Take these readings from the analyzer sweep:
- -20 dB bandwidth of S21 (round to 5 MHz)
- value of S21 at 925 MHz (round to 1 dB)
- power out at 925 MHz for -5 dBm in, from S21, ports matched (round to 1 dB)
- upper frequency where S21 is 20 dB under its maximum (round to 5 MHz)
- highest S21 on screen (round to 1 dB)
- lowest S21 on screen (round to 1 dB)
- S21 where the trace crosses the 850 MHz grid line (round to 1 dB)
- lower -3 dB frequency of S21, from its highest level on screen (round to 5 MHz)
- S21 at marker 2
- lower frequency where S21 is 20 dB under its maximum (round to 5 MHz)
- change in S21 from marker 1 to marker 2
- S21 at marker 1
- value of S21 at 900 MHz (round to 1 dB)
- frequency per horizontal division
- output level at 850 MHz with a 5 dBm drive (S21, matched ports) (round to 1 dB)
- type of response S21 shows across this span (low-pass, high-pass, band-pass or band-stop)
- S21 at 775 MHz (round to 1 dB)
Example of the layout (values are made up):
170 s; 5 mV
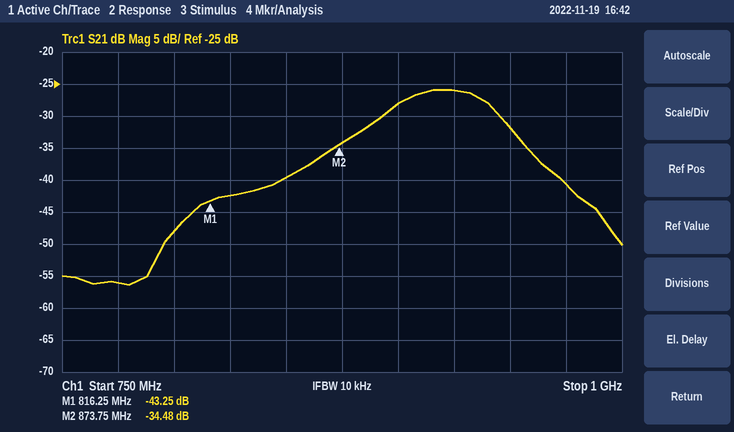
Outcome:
185 MHz; -26 dB; -31 dBm; 990 MHz; -26 dB; -56 dB; -40 dB; 895 MHz; -34.48 dB; 805 MHz; 8.77 dB; -43.25 dB; -28 dB; 25 MHz; -35 dBm; band-pass; -56 dB
